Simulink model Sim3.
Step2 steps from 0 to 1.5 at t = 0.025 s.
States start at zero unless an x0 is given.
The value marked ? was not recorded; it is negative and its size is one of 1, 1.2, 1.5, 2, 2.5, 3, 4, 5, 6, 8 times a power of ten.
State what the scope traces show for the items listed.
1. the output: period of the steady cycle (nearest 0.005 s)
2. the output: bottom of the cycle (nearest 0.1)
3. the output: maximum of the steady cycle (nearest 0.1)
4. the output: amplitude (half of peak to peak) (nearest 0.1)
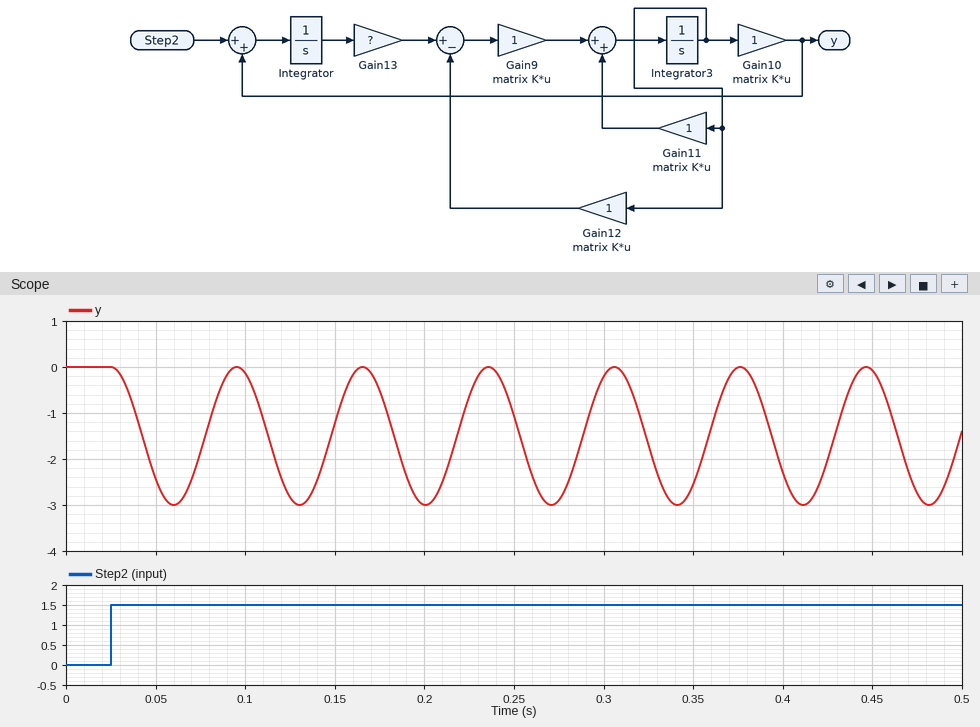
0.070 s
-3.0
0.0
1.5
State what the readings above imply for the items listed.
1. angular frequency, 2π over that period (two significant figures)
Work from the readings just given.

90 rad/s
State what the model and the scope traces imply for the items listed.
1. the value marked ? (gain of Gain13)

-8000
